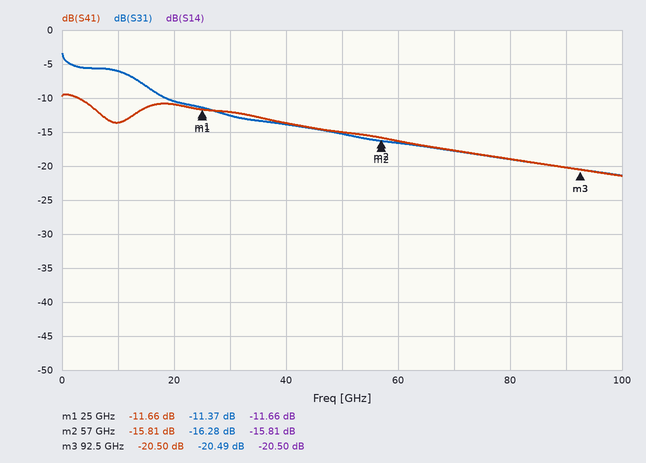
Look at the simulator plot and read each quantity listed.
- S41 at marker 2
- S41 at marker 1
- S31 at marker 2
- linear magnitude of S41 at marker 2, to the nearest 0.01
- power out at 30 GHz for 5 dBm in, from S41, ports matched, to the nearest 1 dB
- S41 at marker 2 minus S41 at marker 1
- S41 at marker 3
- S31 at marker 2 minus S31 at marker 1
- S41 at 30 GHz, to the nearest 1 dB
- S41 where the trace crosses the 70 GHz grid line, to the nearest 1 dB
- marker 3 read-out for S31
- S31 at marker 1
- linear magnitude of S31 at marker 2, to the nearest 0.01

-15.81 dB
-11.66 dB
-16.28 dB
0.16
-7 dBm
-4.15 dB
-20.50 dB
-4.91 dB
-12 dB
-18 dB
-20.49 dB
-11.37 dB
0.15
